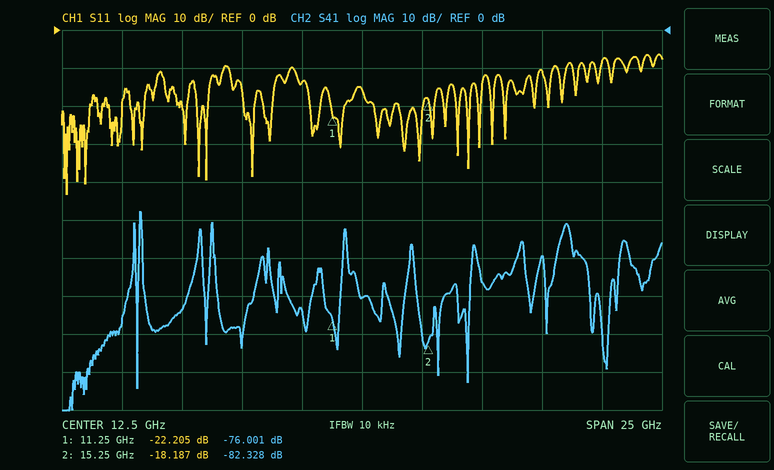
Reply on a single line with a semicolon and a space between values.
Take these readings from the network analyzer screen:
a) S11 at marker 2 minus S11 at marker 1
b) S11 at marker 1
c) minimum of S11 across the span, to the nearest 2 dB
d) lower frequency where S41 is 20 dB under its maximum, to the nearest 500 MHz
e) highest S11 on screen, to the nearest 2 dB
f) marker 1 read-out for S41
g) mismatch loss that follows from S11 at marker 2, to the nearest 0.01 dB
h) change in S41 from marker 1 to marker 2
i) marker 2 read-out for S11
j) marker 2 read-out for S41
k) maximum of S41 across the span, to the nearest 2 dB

4.018 dB; -22.205 dB; -44 dB; 3.0 GHz; -6 dB; -76.001 dB; 0.07 dB; -6.327 dB; -18.187 dB; -82.328 dB; -48 dB
